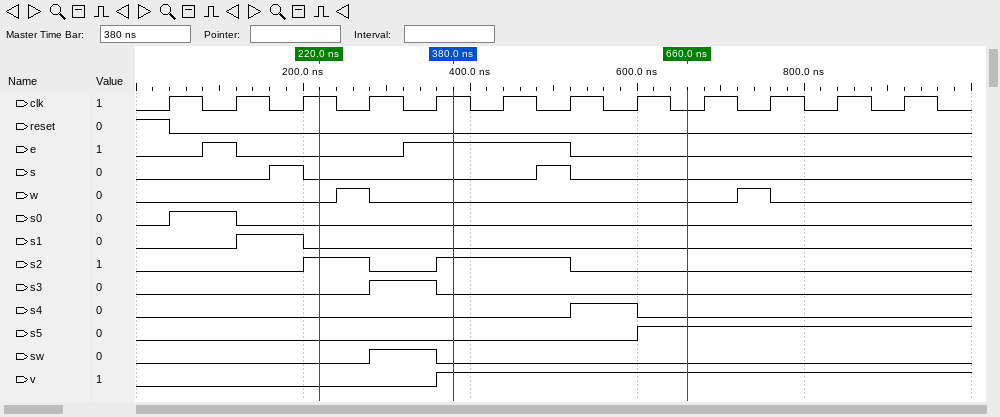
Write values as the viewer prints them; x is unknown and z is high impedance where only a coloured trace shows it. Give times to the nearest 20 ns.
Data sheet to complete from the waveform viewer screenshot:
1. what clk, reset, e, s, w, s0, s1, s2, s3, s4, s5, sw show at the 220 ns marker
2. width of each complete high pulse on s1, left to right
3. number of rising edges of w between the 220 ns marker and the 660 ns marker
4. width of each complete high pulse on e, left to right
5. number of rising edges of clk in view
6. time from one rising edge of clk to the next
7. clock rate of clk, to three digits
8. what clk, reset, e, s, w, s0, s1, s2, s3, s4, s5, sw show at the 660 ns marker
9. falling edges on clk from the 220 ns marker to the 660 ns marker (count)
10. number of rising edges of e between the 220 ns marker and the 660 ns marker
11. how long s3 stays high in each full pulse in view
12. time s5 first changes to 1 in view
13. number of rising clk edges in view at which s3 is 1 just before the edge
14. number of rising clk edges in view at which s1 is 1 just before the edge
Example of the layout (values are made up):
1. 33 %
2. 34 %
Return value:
1. clk=1, reset=0, e=0, s=0, w=0, s0=0, s1=0, s2=1, s3=0, s4=0, s5=0, sw=0
2. 80 ns
3. 1
4. 40 ns, 200 ns
5. 12
6. 80 ns
7. 12.5 MHz
8. clk=0, reset=0, e=0, s=0, w=0, s0=0, s1=0, s2=0, s3=0, s4=0, s5=1, sw=0
9. 6
10. 1
11. 80 ns
12. 600 ns
13. 1
14. 1
